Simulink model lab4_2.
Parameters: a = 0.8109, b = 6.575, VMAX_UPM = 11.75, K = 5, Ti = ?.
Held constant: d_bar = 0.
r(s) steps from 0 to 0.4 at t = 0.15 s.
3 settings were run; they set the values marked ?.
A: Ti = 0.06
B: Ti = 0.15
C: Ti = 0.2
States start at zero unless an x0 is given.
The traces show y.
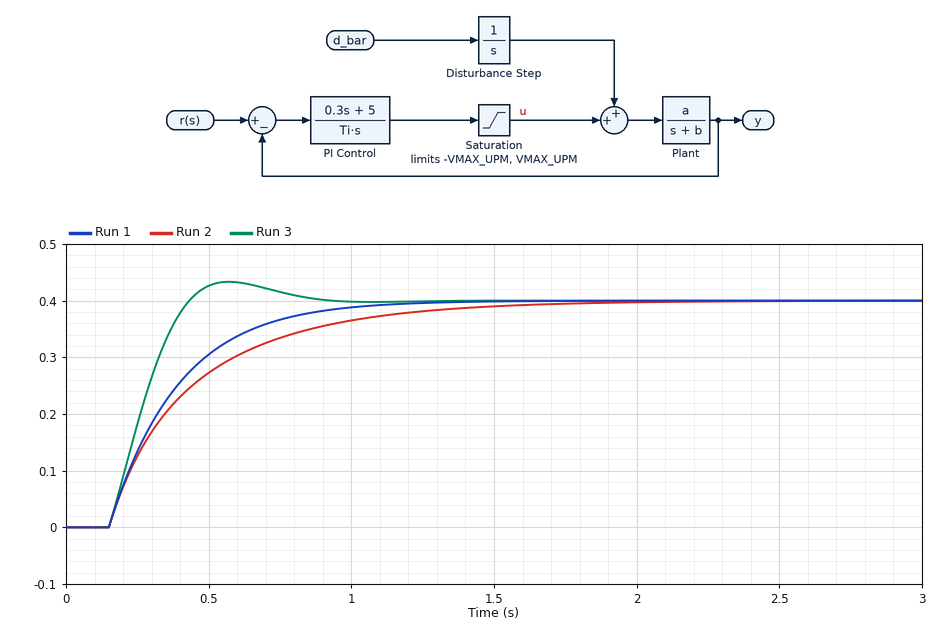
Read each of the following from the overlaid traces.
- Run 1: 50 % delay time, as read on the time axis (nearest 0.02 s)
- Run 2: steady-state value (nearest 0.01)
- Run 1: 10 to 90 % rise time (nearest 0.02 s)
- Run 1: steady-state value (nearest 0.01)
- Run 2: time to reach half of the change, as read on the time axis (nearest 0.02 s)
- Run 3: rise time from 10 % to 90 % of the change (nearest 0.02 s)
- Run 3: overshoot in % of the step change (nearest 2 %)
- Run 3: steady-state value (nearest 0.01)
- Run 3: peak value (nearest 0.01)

0.32 s
0.40
0.54 s
0.40
0.34 s
0.20 s
8 %
0.40
0.43
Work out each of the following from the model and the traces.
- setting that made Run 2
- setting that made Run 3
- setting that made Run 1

C
A
B
